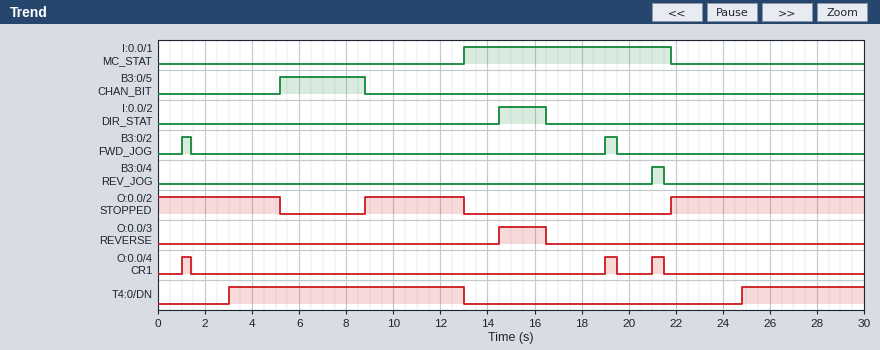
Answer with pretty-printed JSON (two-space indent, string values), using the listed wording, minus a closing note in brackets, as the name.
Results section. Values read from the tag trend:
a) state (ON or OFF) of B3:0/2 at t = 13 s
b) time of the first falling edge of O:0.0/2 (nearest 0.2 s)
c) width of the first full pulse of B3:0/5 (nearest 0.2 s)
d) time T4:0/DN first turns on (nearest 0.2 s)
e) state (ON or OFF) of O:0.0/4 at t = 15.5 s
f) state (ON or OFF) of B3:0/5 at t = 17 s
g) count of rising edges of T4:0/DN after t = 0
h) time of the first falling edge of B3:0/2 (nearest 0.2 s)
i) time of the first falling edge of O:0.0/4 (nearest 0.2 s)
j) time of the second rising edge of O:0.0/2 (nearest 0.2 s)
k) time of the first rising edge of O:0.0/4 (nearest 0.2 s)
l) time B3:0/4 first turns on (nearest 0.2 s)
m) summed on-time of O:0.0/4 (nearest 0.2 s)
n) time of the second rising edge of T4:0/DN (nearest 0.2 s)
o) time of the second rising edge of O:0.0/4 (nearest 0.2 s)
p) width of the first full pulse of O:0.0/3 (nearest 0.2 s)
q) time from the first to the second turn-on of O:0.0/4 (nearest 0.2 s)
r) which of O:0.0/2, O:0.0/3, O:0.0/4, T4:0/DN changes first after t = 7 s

{
  "state (ON or OFF) of B3:0/2 at t = 13 s": "OFF",
  "time of the first falling edge of O:0.0/2": "5.2 s",
  "width of the first full pulse of B3:0/5": "3.6 s",
  "time T4:0/DN first turns on": "3.0 s",
  "state (ON or OFF) of O:0.0/4 at t = 15.5 s": "OFF",
  "state (ON or OFF) of B3:0/5 at t = 17 s": "OFF",
  "count of rising edges of T4:0/DN after t = 0": "2",
  "time of the first falling edge of B3:0/2": "1.4 s",
  "time of the first falling edge of O:0.0/4": "1.4 s",
  "time of the second rising edge of O:0.0/2": "21.8 s",
  "time of the first rising edge of O:0.0/4": "1.0 s",
  "time B3:0/4 first turns on": "21.0 s",
  "summed on-time of O:0.0/4": "1.4 s",
  "time of the second rising edge of T4:0/DN": "24.8 s",
  "time of the second rising edge of O:0.0/4": "19.0 s",
  "width of the first full pulse of O:0.0/3": "2.0 s",
  "time from the first to the second turn-on of O:0.0/4": "18.0 s",
  "which of O:0.0/2, O:0.0/3, O:0.0/4, T4:0/DN changes first after t = 7 s": "O:0.0/2"
}
